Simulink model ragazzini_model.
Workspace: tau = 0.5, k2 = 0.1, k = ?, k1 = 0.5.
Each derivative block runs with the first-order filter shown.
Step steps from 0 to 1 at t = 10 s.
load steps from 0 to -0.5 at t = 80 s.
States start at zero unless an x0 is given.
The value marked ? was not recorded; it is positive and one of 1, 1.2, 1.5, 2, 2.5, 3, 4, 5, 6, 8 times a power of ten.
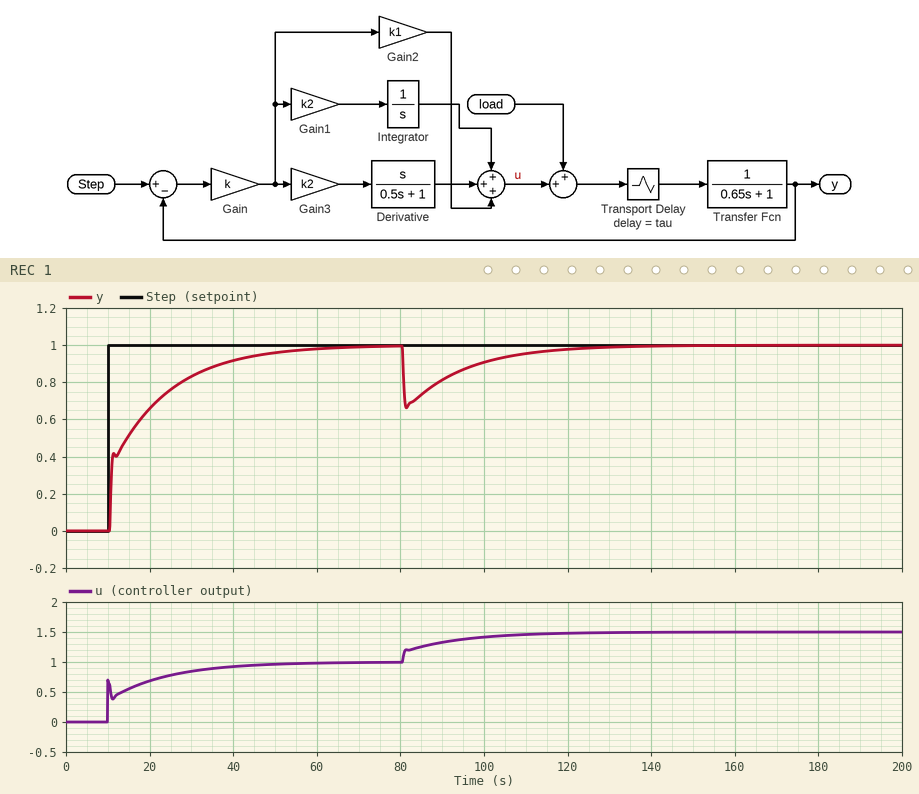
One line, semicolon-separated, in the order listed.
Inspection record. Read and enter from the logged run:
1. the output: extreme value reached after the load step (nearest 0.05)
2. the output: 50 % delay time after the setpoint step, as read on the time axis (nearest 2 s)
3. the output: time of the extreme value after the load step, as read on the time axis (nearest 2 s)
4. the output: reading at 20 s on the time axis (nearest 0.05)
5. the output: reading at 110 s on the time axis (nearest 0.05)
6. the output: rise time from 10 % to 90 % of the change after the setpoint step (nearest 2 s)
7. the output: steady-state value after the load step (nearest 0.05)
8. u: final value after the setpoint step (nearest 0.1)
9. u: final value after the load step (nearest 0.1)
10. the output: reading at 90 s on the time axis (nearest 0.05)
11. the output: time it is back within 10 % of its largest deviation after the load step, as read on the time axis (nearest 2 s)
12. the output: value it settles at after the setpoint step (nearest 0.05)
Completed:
0.65; 14 s; 82 s; 0.65; 0.95; 26 s; 1.00; 1.0; 1.5; 0.80; 114 s; 1.00
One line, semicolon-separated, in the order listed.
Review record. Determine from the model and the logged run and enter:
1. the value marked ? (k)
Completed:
1
